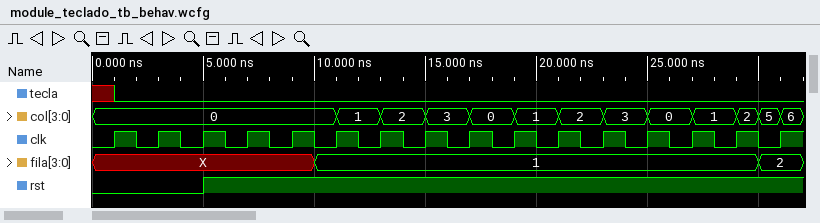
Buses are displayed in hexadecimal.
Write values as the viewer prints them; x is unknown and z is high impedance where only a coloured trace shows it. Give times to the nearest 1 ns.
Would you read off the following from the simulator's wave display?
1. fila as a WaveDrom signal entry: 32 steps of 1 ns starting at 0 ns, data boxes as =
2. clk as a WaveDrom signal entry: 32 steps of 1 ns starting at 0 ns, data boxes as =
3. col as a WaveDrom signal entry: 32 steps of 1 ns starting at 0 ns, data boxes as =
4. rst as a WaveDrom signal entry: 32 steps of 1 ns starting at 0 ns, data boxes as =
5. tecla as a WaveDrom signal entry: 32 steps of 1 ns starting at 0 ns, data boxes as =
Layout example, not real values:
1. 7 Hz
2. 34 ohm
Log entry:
1. {name: 'fila', wave: 'x.........=...................=.', data: '1 2'}
2. {name: 'clk', wave: '01010101010101010101010101010101'}
3. {name: 'col', wave: '=..........=.=.=.=.=.=.=.=.=.===', data: '0 1 2 3 0 1 2 3 0 1 2 5 6'}
4. {name: 'rst', wave: '0....1..........................'}
5. {name: 'tecla', wave: 'x0..............................'}
